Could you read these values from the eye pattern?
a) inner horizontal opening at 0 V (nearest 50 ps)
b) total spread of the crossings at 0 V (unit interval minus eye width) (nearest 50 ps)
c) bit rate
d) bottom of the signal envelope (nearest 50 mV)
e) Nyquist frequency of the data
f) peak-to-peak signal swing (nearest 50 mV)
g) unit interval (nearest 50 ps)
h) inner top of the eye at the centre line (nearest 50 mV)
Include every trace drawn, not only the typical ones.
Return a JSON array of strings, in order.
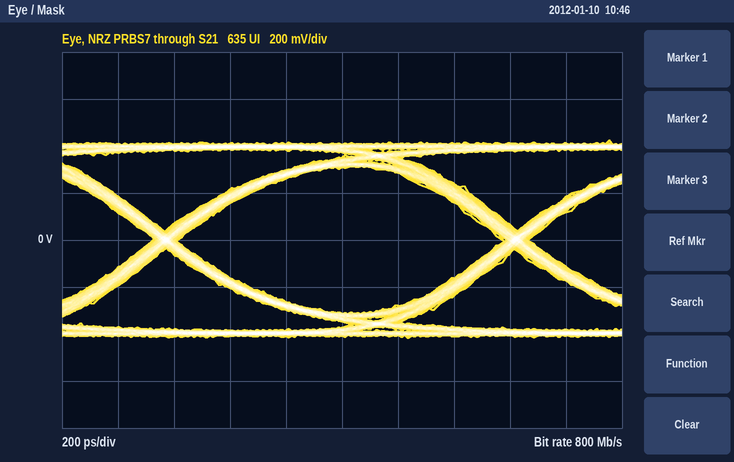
["1.15 ns", "100 ps", "800 Mb/s", "-400 mV", "400 MHz", "850 mV", "1.25 ns", "300 mV"]
